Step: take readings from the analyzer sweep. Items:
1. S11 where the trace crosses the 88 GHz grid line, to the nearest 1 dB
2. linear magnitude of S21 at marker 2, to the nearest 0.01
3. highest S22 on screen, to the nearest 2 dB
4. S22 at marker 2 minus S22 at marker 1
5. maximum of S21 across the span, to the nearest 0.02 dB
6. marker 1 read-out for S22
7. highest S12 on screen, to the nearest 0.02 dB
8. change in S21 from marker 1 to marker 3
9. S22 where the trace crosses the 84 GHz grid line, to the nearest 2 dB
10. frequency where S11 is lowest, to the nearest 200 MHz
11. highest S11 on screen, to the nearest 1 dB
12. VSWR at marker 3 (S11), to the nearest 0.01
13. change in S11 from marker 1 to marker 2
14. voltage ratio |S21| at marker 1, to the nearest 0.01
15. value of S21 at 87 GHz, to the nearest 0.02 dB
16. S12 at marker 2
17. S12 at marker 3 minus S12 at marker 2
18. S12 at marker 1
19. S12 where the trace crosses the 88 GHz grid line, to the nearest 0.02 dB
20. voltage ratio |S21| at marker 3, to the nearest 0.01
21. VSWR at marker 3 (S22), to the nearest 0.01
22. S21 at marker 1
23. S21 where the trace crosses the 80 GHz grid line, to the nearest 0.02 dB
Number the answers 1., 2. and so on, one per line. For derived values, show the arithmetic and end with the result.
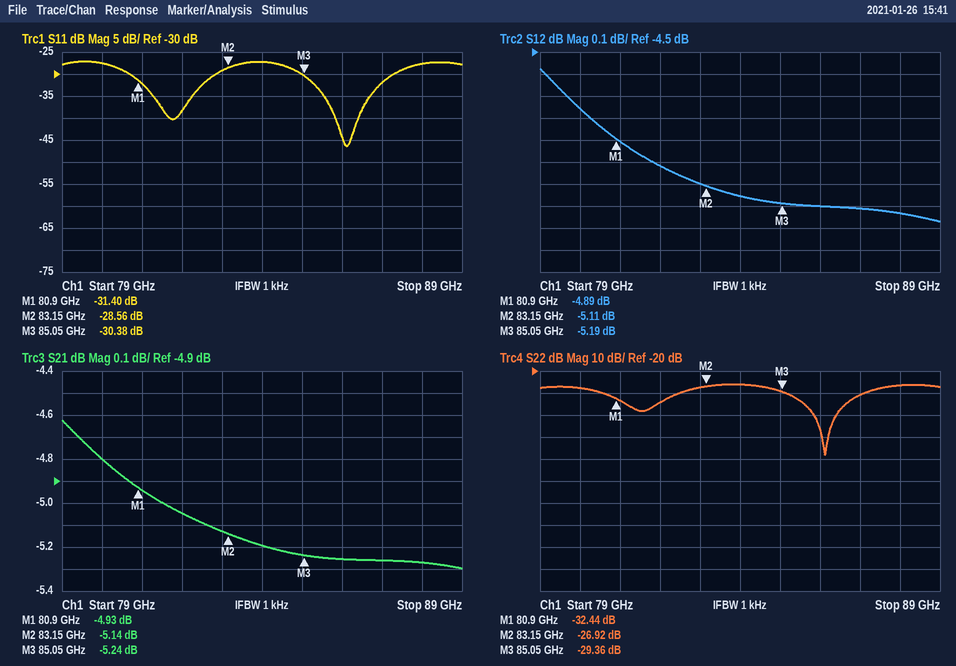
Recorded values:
1. -28 dB
2. 10^(-5.14/20) ≈ 0.55
3. -26 dB
4. -26.92 − (-32.44) = 5.52 dB
5. -4.62 dB
6. -32.44 dB
7. -4.58 dB
8. -5.24 − (-4.93) = -0.31 dB
9. -26 dB
10. 86.2 GHz
11. -27 dB
12. (1 + 0.0303)/(1 − 0.0303) ≈ 1.06
13. -28.56 − (-31.4) = 2.84 dB
14. 10^(-4.93/20) ≈ 0.57
15. -5.26 dB
16. -5.11 dB
17. -5.19 − (-5.11) = -0.08 dB
18. -4.89 dB
19. -5.24 dB
20. 10^(-5.24/20) ≈ 0.55
21. (1 + 0.0340)/(1 − 0.0340) ≈ 1.07
22. -4.93 dB
23. -4.80 dB
